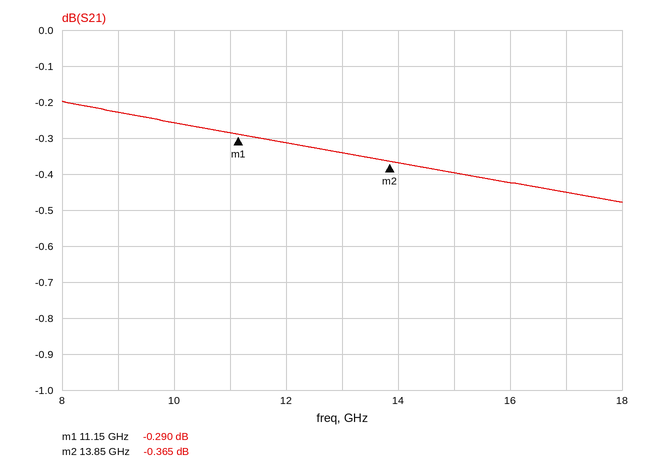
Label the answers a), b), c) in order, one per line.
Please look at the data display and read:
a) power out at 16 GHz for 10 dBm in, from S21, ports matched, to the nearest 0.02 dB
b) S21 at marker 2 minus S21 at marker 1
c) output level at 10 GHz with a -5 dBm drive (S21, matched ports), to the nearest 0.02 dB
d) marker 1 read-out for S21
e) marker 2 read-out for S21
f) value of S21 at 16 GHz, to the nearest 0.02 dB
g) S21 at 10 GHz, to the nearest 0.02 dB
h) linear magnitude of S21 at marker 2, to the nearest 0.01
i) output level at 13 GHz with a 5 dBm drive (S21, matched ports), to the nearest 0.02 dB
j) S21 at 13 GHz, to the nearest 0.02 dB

a) 9.58 dBm
b) -0.075 dB
c) -5.26 dBm
d) -0.290 dB
e) -0.365 dB
f) -0.42 dB
g) -0.26 dB
h) 0.96
i) 4.66 dBm
j) -0.34 dB
